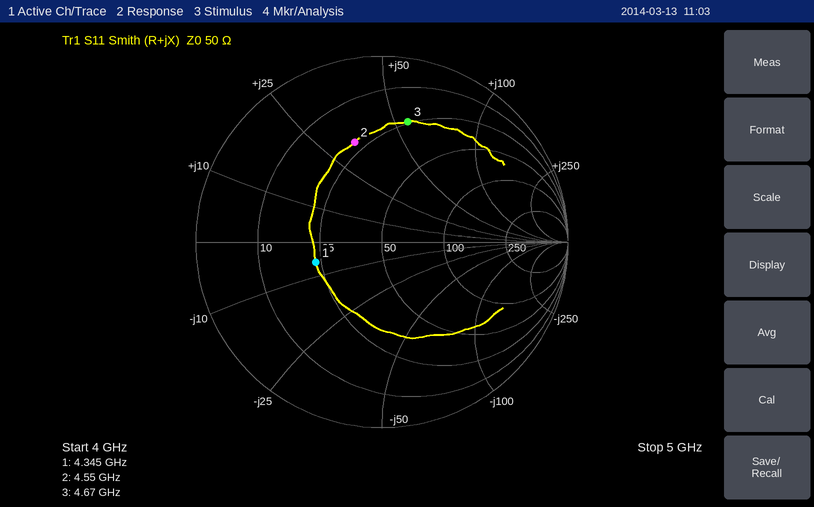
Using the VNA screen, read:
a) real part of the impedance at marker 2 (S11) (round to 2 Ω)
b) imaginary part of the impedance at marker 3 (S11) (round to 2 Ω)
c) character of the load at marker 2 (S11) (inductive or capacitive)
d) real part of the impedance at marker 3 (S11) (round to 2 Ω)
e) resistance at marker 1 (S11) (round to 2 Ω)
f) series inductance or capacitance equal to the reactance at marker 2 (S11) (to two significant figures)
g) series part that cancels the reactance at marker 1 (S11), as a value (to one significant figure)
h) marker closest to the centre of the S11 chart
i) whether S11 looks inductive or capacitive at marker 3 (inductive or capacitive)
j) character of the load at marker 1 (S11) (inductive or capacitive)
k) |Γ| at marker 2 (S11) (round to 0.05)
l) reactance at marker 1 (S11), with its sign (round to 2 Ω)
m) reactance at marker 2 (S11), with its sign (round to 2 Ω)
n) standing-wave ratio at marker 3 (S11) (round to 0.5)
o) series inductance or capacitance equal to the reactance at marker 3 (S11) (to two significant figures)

22 Ω
+56 Ω
inductive
24 Ω
24 Ω
1.2 nH
200 pH
marker 1
inductive
capacitive
0.55
-6 Ω
+34 Ω
5.0
1.9 nH
